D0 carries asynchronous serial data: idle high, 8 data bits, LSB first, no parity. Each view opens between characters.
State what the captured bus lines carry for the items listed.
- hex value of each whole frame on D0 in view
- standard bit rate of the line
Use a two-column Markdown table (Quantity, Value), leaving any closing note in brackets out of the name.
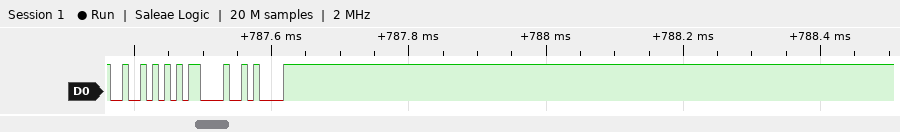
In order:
| Quantity | Value |
|---|---|
| hex value of each whole frame on D0 in view | 52, 0D, 0A |
| standard bit rate of the line | 115200 baud |
